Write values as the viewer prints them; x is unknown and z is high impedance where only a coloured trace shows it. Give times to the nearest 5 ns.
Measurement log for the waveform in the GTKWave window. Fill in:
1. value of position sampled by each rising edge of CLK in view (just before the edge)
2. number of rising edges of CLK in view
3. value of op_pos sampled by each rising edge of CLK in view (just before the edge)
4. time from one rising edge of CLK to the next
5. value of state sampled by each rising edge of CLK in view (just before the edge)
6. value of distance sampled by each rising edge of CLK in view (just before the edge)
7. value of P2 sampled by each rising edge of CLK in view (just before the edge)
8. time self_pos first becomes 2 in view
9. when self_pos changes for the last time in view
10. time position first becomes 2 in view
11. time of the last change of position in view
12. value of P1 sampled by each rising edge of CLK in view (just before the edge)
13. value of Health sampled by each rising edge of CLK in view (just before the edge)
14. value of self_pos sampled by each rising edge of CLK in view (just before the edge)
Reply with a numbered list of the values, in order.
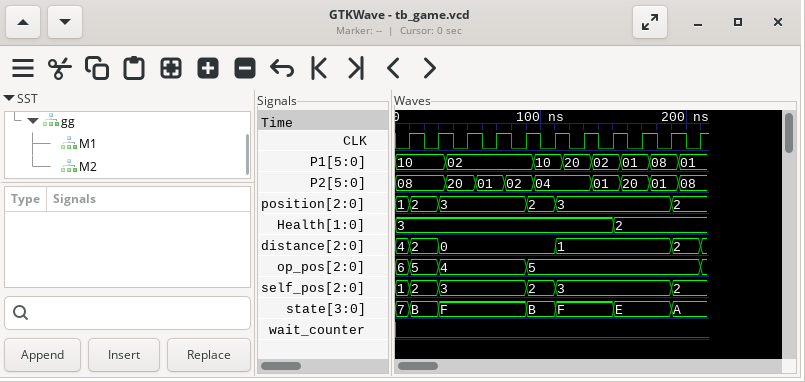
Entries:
1. 1, 2, 3, 3, 3, 2, 3, 3, 3, 3, 2
2. 11
3. 6, 5, 4, 4, 4, 5, 5, 5, 5, 5, 5
4. 20 ns
5. 7, B, F, F, F, B, F, F, E, E, A
6. 4, 2, 0, 0, 0, 0, 1, 1, 1, 1, 2
7. 08, 08, 20, 01, 02, 04, 04, 01, 20, 01, 08
8. 10 ns
9. 190 ns
10. 10 ns
11. 190 ns
12. 10, 10, 02, 02, 02, 10, 20, 02, 01, 08, 01
13. 3, 3, 3, 3, 3, 3, 3, 3, 2, 2, 2
14. 1, 2, 3, 3, 3, 2, 3, 3, 3, 3, 2
